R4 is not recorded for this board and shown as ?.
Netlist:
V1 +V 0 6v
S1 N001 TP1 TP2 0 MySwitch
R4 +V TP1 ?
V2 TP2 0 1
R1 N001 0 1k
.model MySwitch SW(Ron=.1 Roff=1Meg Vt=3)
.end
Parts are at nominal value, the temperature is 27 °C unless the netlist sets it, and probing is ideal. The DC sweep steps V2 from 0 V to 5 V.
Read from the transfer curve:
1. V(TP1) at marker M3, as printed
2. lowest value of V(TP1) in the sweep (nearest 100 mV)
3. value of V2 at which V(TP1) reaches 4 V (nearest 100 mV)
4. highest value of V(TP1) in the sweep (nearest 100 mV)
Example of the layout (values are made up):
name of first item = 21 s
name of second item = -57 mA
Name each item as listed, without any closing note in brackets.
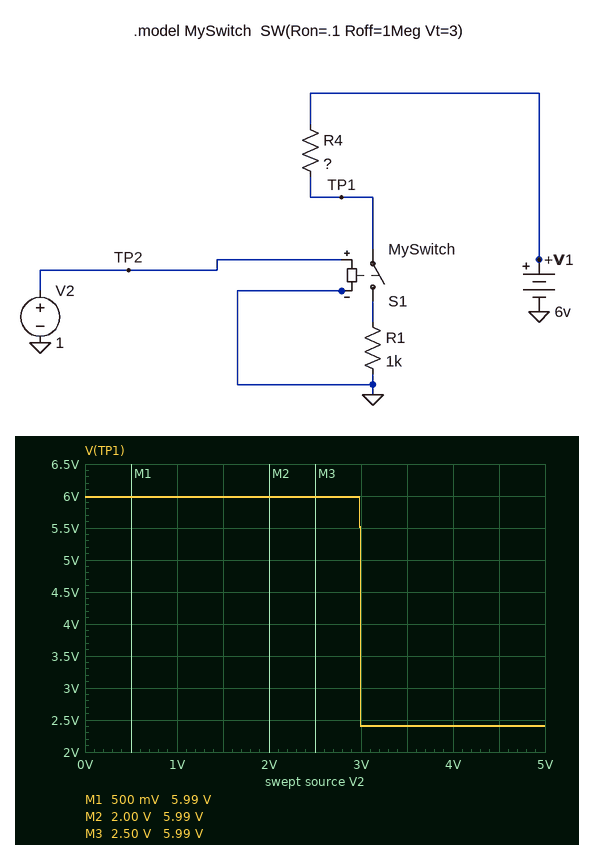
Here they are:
V(TP1) at marker M3, as printed = 5.99 V
lowest value of V(TP1) in the sweep = 2.4 V
value of V2 at which V(TP1) reaches 4 V = 3.0 V
highest value of V(TP1) in the sweep = 6.0 V
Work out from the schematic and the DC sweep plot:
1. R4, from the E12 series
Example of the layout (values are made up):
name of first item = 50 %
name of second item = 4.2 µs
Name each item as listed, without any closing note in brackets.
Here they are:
R4, from the E12 series = 1.5 kΩ
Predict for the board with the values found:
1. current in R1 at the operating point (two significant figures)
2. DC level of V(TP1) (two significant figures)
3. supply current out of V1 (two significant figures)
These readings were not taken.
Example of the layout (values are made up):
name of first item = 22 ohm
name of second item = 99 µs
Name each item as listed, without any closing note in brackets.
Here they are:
current in R1 at the operating point = 6.0 µA
DC level of V(TP1) = 6.0 V
supply current out of V1 = 6.0 µA
